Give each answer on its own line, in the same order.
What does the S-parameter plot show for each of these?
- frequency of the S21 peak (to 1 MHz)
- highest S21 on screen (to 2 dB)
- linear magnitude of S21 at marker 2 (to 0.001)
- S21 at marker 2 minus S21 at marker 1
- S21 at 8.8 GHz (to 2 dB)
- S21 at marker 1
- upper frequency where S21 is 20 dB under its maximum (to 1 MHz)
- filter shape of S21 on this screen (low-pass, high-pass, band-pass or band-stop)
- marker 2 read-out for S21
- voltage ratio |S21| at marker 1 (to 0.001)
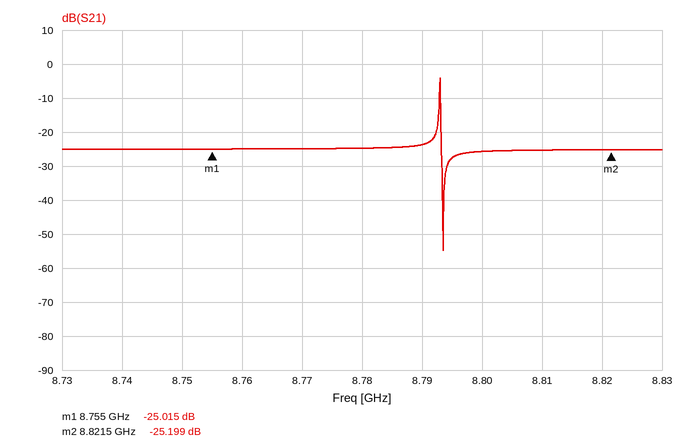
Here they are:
8.793 GHz
-4 dB
0.055
-0.184 dB
-26 dB
-25.015 dB
8.793 GHz
band-pass
-25.199 dB
0.056
